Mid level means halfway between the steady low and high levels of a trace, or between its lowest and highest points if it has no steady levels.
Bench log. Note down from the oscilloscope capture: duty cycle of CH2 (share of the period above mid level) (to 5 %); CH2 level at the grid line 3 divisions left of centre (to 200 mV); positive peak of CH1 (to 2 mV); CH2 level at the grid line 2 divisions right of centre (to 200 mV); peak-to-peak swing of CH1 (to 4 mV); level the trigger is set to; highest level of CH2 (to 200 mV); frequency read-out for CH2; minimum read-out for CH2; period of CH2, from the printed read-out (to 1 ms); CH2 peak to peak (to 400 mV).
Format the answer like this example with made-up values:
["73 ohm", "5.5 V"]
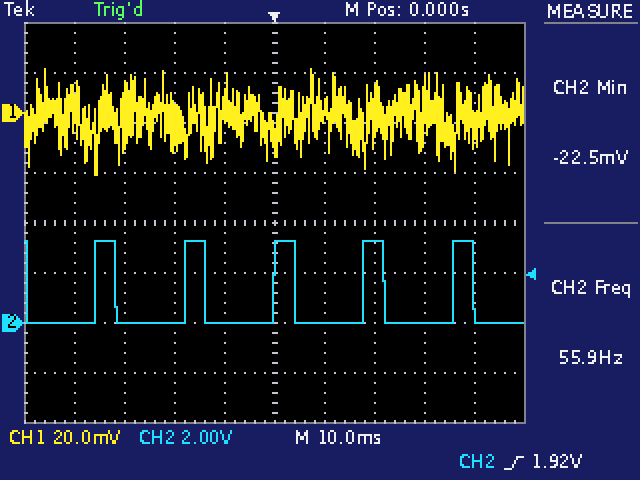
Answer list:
["25 %", "0.0 V", "18 mV", "3.2 V", "44 mV", "1.92 V", "3.2 V", "55.9 Hz", "-22.5 mV", "18 ms", "3.2 V"]
